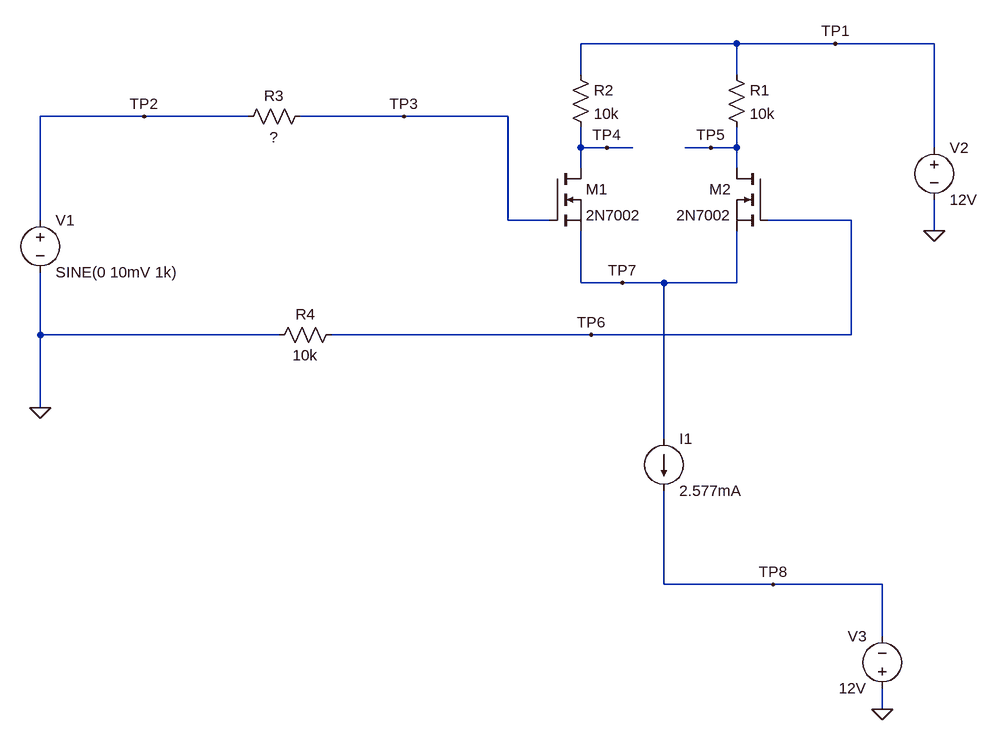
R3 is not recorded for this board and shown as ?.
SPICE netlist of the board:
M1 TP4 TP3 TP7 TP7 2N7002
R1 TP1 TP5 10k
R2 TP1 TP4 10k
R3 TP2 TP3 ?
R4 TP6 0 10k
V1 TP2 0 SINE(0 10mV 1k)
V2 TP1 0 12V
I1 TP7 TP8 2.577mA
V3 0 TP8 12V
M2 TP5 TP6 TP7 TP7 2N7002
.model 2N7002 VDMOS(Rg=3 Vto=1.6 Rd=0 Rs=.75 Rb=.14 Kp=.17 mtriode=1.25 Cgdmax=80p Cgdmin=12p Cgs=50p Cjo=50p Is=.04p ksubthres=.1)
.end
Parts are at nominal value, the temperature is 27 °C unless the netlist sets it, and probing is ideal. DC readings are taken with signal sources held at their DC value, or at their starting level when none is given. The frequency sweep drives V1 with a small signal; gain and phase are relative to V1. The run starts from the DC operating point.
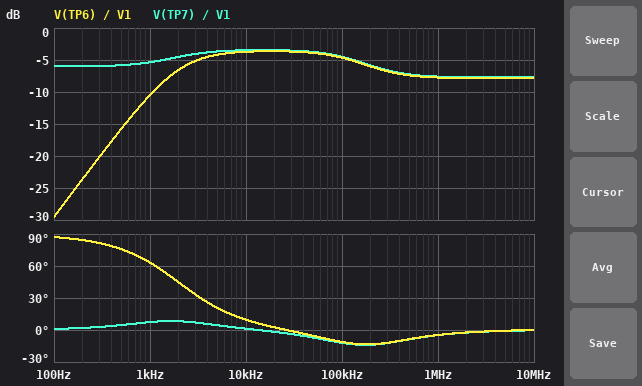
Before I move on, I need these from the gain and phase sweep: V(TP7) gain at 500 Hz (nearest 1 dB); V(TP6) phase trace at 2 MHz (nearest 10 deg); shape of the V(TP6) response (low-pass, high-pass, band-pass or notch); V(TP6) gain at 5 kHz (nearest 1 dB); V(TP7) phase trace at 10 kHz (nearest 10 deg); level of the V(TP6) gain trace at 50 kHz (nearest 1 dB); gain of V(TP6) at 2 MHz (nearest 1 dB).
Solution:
-6 dB
0 deg
high-pass
-4 dB
0 deg
-4 dB
-8 dB
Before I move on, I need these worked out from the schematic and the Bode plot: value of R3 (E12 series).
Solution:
4.7 kΩ
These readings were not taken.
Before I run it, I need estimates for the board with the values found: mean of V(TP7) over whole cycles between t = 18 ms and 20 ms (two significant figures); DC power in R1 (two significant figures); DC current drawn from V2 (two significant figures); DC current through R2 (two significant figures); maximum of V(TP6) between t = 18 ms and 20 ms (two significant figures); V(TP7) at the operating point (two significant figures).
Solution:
-1.7 V
17 mW
2.6 mA
1.3 mA
3.0 mV
-1.7 V
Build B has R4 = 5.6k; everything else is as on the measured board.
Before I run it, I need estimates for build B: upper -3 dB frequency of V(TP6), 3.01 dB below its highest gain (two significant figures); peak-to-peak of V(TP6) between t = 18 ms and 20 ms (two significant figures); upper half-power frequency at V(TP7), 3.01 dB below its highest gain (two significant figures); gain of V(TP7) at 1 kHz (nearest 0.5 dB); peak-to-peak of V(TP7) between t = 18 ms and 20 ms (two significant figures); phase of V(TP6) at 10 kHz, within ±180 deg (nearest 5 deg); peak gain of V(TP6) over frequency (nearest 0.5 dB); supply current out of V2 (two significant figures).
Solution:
460 kHz
3.5 mV
420 kHz
-6.0 dB
10 mV
15 deg
-5.5 dB
2.6 mA
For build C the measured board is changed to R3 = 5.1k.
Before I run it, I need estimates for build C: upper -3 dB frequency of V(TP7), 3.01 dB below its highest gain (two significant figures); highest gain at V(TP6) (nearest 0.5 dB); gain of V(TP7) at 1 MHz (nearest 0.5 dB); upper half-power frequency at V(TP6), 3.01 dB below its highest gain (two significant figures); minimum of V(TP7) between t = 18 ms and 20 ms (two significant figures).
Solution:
250 kHz
-4.0 dB
-8.0 dB
260 kHz
-1.7 V
